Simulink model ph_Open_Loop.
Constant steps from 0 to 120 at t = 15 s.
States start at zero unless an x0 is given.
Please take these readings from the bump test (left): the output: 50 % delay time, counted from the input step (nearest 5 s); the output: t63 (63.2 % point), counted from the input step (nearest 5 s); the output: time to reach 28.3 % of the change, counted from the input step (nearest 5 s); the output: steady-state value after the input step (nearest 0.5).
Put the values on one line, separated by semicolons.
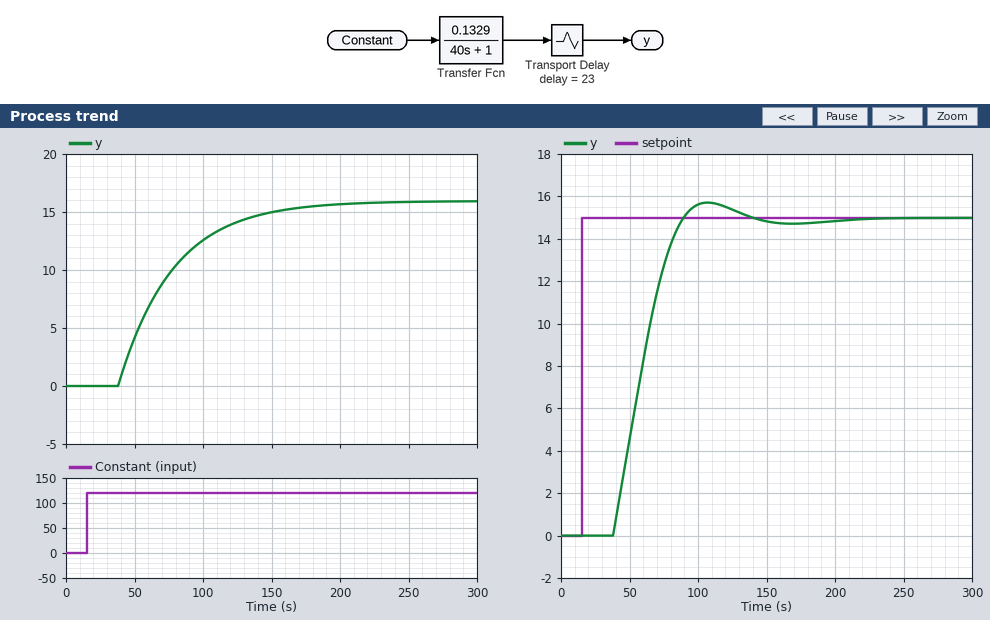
50 s; 65 s; 35 s; 16.0
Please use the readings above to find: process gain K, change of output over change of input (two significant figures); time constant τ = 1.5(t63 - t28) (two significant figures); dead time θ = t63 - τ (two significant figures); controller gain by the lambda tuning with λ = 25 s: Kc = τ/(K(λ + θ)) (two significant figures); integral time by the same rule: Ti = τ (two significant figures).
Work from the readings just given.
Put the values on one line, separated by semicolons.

0.13; 45 s; 20 s; 7.7; 45 s
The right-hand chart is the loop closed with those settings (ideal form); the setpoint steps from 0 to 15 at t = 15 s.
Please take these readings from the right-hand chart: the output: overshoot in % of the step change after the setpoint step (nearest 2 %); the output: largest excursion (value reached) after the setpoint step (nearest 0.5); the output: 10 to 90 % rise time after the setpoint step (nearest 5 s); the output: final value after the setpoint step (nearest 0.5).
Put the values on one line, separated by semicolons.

4 %; 15.5; 35 s; 15.0
